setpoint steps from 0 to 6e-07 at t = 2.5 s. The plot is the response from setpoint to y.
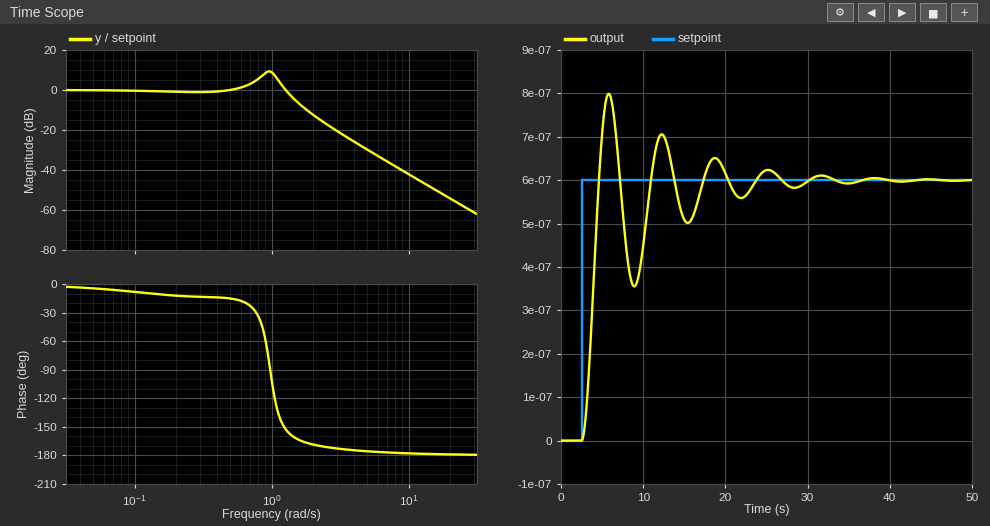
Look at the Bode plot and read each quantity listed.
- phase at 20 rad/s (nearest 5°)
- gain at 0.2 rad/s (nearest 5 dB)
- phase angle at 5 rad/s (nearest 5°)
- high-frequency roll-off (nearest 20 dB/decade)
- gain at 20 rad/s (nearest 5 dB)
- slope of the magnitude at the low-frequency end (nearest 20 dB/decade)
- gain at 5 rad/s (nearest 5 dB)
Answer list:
-180°
0 dB
-175°
-40 dB/decade
-55 dB
0 dB/decade
-30 dB
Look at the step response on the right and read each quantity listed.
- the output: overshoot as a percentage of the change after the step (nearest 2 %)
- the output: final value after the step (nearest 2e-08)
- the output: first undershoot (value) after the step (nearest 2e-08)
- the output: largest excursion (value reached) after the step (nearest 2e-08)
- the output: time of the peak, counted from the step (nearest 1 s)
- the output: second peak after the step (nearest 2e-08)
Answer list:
34 %
0.00000060
0.00000036
0.00000080
3 s
0.00000070
